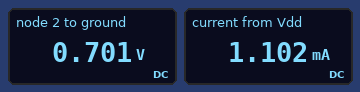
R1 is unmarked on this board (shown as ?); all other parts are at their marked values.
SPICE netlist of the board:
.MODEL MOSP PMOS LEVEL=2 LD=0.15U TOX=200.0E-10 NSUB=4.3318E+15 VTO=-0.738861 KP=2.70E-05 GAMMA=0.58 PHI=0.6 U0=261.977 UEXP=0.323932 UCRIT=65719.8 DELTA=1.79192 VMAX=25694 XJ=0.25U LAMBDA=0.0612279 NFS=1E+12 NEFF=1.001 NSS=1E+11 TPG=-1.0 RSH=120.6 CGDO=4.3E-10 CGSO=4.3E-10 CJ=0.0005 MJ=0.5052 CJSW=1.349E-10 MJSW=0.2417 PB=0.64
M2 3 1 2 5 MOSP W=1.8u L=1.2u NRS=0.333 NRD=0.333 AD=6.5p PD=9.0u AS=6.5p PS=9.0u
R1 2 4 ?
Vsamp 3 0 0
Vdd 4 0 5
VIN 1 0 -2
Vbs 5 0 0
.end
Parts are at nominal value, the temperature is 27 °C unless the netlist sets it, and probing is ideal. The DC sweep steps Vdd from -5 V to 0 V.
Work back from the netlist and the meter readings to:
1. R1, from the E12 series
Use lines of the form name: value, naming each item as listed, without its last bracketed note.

R1, from the E12 series: 3.9 kΩ
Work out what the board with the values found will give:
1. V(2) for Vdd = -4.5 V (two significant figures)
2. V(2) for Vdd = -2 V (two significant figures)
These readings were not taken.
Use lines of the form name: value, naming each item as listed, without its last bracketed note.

V(2) for Vdd = -4.5 V: -4.4 V
V(2) for Vdd = -2 V: -1.9 V
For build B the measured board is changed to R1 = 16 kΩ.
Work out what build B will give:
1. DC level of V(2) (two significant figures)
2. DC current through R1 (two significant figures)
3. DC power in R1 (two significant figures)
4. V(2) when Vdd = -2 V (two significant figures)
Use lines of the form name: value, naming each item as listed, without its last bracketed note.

DC level of V(2): 630 mV
DC current through R1: 270 µA
DC power in R1: 1.2 mW
V(2) when Vdd = -2 V: -1.6 V
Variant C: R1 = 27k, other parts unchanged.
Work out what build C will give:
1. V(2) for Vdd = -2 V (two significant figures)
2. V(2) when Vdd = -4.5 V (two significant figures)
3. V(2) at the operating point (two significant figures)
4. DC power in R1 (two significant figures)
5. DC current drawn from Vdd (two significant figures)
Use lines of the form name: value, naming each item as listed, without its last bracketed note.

V(2) for Vdd = -2 V: -1.3 V
V(2) when Vdd = -4.5 V: -3.6 V
V(2) at the operating point: 610 mV
DC power in R1: 710 µW
DC current drawn from Vdd: 160 µA
